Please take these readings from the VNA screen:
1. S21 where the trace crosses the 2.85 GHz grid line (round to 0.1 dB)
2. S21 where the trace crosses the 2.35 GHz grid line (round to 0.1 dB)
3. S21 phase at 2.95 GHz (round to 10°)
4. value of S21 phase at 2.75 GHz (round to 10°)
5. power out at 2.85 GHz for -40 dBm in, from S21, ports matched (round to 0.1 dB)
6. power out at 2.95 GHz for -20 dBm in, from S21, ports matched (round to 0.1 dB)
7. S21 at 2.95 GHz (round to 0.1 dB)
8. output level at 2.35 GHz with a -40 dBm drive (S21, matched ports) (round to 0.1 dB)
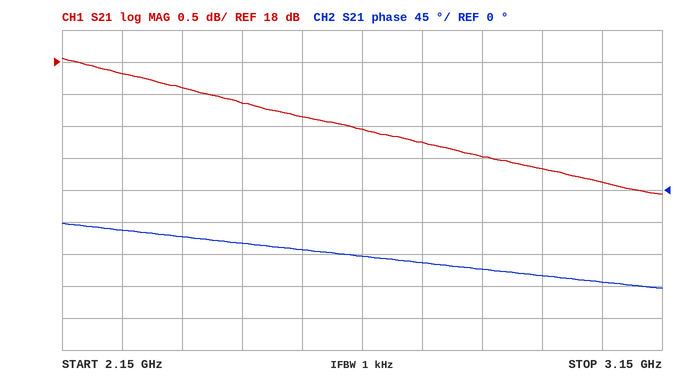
16.5 dB
17.6 dB
-120°
-100°
-23.5 dBm
-3.7 dBm
16.3 dB
-22.4 dBm
